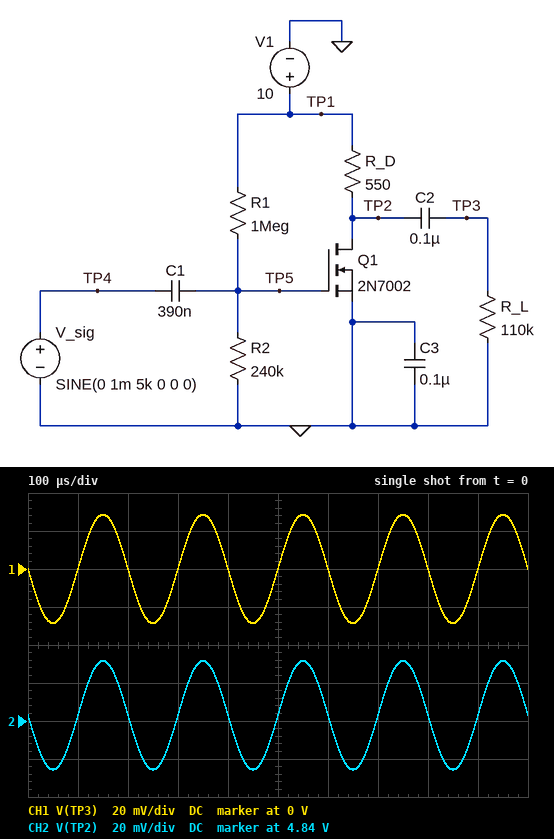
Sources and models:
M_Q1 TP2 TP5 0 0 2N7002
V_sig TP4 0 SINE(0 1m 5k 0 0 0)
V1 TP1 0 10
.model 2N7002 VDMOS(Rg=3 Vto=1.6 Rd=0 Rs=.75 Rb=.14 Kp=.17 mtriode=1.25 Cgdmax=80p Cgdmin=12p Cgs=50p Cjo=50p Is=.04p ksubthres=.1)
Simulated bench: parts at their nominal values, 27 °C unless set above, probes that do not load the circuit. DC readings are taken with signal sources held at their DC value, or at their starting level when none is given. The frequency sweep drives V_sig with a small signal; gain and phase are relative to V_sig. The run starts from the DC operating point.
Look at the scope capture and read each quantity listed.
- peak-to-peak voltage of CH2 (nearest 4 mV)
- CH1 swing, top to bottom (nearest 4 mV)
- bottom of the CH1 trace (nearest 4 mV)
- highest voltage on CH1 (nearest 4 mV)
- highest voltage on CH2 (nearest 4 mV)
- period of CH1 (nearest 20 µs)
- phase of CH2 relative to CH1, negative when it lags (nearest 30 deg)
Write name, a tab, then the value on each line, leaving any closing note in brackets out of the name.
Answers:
peak-to-peak voltage of CH2	56 mV
CH1 swing, top to bottom	56 mV
bottom of the CH1 trace	-28 mV
highest voltage on CH1	28 mV
highest voltage on CH2	4.872 V
period of CH1	200 µs
phase of CH2 relative to CH1, negative when it lags	0 deg
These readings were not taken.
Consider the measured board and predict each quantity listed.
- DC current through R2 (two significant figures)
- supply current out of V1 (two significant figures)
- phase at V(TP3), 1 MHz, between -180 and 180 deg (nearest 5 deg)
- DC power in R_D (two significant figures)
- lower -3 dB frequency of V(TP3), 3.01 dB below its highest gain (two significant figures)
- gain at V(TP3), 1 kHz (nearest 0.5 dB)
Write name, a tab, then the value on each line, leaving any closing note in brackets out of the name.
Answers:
DC current through R2	8.1 µA
supply current out of V1	9.4 mA
phase at V(TP3), 1 MHz, between -180 and 180 deg	170 deg
DC power in R_D	48 mW
lower -3 dB frequency of V(TP3), 3.01 dB below its highest gain	15 Hz
gain at V(TP3), 1 kHz	29.0 dB
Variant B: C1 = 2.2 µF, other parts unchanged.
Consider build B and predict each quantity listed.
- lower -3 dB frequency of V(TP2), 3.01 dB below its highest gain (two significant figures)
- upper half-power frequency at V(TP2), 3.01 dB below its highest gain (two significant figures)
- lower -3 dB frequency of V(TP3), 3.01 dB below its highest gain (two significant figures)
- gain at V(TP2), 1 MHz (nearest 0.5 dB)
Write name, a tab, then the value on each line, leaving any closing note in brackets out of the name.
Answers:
lower -3 dB frequency of V(TP2), 3.01 dB below its highest gain	370 mHz
upper half-power frequency at V(TP2), 3.01 dB below its highest gain	6.7 MHz
lower -3 dB frequency of V(TP3), 3.01 dB below its highest gain	14 Hz
gain at V(TP2), 1 MHz	29.0 dB
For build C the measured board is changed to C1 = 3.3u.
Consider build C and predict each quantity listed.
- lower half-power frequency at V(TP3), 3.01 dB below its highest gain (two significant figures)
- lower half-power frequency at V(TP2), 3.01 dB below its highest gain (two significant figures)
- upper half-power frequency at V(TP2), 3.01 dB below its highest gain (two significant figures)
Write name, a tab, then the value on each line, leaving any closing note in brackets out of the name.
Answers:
lower half-power frequency at V(TP3), 3.01 dB below its highest gain	14 Hz
lower half-power frequency at V(TP2), 3.01 dB below its highest gain	250 mHz
upper half-power frequency at V(TP2), 3.01 dB below its highest gain	6.7 MHz
